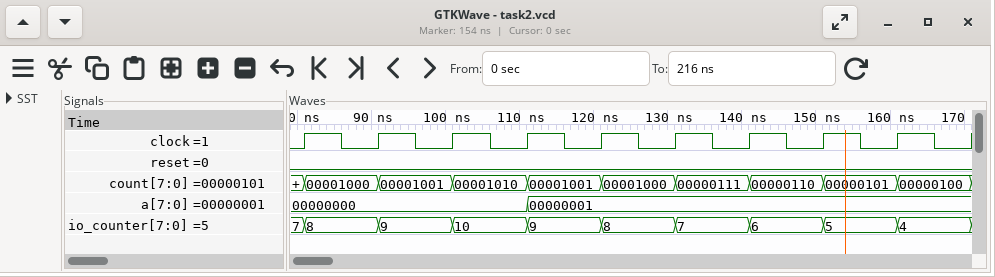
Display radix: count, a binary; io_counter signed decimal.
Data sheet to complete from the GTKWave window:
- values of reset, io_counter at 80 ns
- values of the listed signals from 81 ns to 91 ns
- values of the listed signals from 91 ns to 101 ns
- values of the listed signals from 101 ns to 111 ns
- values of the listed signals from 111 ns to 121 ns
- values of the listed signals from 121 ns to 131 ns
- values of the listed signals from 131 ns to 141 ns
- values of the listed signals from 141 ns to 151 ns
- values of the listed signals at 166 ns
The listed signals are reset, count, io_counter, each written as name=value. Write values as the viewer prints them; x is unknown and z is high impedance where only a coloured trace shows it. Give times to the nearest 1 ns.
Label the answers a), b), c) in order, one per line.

a) reset=0, io_counter=7
b) reset=0, count=00001000, io_counter=8
c) reset=0, count=00001001, io_counter=9
d) reset=0, count=00001010, io_counter=10
e) reset=0, count=00001001, io_counter=9
f) reset=0, count=00001000, io_counter=8
g) reset=0, count=00000111, io_counter=7
h) reset=0, count=00000110, io_counter=6
i) reset=0, count=00000100, io_counter=4
